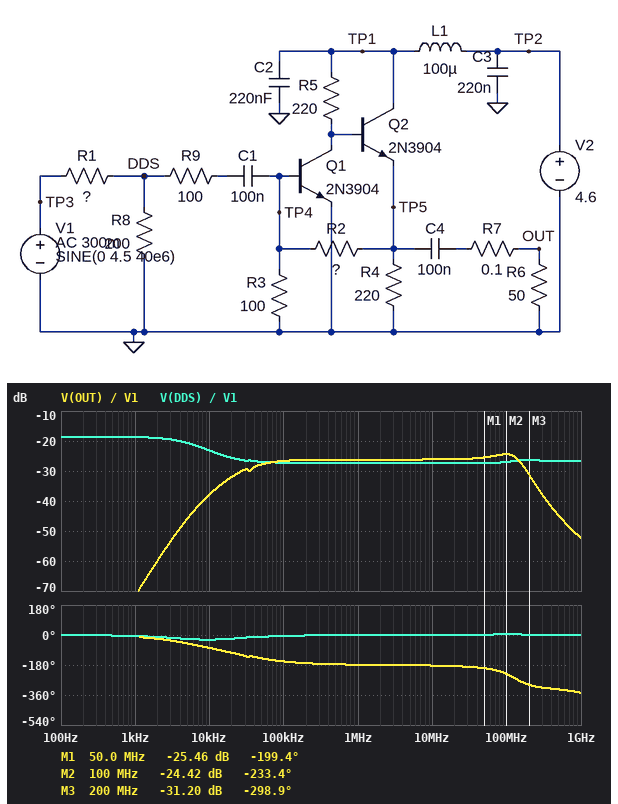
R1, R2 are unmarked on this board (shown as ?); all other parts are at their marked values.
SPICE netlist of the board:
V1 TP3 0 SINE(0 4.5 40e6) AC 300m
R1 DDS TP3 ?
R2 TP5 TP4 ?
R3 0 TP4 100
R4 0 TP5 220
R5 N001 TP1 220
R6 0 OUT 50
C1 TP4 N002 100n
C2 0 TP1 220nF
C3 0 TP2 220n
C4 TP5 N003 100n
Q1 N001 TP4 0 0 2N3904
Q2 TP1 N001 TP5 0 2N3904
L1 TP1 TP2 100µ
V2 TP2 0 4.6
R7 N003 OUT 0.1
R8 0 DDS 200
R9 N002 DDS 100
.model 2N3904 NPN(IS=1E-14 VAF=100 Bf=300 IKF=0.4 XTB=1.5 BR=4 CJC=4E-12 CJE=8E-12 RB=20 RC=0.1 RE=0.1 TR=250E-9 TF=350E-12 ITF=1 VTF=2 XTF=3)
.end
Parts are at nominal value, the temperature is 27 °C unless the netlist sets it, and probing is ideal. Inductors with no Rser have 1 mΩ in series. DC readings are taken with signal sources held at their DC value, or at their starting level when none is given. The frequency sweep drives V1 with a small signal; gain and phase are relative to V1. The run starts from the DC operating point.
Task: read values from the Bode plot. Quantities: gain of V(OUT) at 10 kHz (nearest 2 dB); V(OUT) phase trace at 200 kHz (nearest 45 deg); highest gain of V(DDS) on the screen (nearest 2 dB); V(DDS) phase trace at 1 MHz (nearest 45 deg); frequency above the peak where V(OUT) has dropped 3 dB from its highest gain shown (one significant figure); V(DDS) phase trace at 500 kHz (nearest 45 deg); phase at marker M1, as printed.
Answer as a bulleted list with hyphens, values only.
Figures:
- -38 dB
- -180 deg
- -18 dB
- 0 deg
- 200 MHz
- 0 deg
- -199.4 deg
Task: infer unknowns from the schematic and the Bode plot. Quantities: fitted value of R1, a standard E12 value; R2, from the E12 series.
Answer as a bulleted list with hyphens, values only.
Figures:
- 1.5 kΩ
- 120 Ω
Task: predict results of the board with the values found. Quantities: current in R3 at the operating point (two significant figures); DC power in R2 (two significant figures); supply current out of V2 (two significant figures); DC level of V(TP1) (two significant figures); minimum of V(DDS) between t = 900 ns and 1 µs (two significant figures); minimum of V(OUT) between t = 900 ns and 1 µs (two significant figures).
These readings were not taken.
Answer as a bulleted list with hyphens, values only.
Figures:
- 7.2 mA
- 6.2 mW
- 25 mA
- 4.6 V
- -190 mV
- -230 mV
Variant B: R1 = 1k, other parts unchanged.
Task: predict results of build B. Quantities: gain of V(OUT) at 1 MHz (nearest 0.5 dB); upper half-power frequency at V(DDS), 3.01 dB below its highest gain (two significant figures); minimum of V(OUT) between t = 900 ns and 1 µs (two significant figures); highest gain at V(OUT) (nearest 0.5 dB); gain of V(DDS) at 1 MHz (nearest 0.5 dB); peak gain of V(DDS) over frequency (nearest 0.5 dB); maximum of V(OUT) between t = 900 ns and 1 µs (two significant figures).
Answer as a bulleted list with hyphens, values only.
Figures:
- -23.0 dB
- 7.0 kHz
- -340 mV
- -21.0 dB
- -24.0 dB
- -15.5 dB
- 340 mV
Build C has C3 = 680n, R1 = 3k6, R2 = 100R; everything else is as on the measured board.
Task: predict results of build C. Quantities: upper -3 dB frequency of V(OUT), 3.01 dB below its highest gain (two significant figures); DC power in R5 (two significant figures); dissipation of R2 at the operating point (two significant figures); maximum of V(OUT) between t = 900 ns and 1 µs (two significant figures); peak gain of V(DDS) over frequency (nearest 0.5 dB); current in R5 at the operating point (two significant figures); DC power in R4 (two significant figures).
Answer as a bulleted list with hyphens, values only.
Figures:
- 170 MHz
- 27 mW
- 5.2 mW
- 83 mV
- -25.5 dB
- 11 mA
- 9.5 mW
